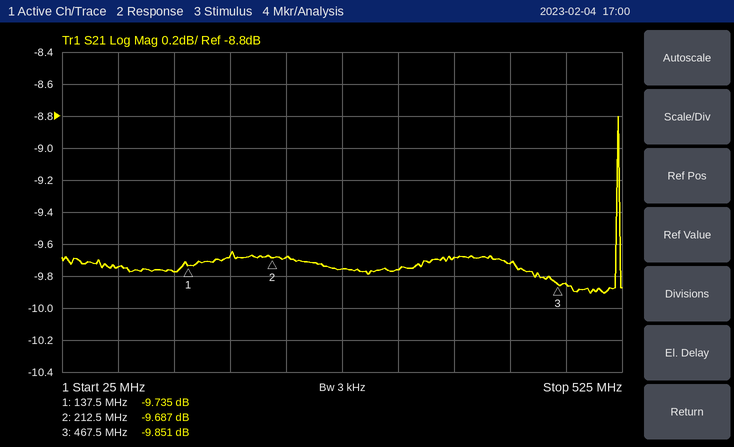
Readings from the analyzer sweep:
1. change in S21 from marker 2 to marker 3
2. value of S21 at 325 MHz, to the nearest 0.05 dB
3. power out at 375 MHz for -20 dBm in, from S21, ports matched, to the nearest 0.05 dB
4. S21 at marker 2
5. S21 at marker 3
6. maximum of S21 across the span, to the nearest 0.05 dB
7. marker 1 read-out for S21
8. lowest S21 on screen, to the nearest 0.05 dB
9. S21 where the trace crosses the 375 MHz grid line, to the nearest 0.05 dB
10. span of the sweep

-0.164 dB
-9.75 dB
-29.70 dBm
-9.687 dB
-9.851 dB
-8.80 dB
-9.735 dB
-9.90 dB
-9.70 dB
500 MHz
